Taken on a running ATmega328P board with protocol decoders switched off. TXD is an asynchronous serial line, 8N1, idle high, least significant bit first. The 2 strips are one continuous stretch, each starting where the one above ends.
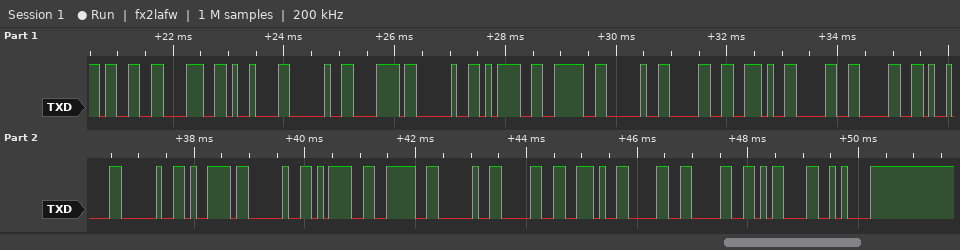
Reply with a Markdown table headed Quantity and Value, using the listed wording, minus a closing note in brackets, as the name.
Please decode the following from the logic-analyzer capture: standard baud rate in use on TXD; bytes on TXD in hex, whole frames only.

| Quantity | Value |
|---|---|
| standard baud rate in use on TXD | 9600 baud |
| bytes on TXD in hex, whole frames only | 33 38 09 20 78 20 3D 3E 20 30 2E 30 30 09 20 79 20 3D 3E 20 30 2E 30 30 0D 0A |
